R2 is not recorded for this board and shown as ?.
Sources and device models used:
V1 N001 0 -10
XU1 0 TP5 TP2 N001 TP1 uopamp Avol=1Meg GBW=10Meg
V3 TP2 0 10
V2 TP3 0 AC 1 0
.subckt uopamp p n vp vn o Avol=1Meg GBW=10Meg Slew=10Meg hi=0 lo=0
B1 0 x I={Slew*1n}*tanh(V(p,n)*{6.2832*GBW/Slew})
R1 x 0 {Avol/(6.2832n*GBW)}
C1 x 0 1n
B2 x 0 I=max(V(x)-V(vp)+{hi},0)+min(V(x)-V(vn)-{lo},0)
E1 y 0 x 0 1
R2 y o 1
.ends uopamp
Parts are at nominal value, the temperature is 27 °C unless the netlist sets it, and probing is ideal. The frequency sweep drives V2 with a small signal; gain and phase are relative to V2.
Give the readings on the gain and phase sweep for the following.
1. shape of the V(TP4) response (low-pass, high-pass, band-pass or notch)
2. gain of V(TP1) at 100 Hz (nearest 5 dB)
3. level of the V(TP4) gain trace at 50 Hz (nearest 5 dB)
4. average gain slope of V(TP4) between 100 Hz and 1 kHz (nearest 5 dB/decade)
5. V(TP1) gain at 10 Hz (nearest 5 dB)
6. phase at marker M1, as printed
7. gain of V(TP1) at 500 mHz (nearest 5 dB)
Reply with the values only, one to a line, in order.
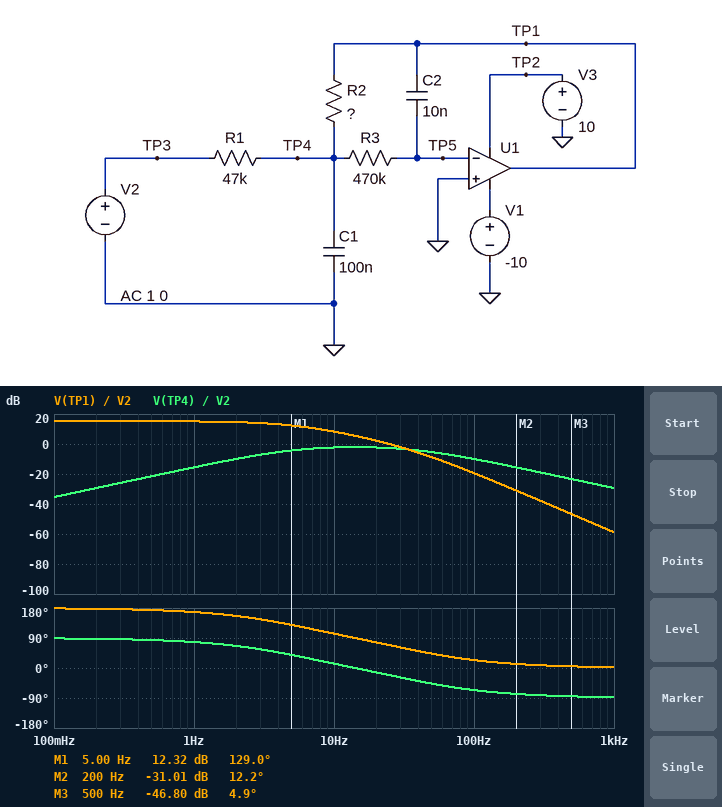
band-pass
-20 dB
-5 dB
-20 dB/decade
10 dB
129.0 deg
15 dB
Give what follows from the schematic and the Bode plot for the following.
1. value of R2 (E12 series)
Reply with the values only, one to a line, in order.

270 kΩ
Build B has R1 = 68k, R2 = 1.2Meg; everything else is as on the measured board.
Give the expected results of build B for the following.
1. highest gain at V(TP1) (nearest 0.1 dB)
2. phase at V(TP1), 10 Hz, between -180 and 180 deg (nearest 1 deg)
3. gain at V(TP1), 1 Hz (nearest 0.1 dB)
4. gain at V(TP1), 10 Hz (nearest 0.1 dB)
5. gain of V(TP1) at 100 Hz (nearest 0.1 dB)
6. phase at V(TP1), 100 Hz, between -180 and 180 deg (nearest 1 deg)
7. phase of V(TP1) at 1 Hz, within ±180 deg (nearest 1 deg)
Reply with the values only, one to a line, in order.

24.9 dB
79 deg
23.6 dB
8.8 dB
-22.3 dB
16 deg
147 deg
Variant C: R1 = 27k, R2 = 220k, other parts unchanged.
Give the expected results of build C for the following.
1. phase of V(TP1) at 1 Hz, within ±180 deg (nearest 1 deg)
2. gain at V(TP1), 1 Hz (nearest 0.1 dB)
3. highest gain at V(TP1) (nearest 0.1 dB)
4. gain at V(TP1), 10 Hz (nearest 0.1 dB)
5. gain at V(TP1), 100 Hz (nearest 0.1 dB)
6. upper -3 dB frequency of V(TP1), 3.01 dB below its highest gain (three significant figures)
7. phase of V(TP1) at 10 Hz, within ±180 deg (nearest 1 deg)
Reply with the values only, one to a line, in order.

164 deg
17.9 dB
18.2 dB
9.0 dB
-15.6 dB
3.71 Hz
102 deg
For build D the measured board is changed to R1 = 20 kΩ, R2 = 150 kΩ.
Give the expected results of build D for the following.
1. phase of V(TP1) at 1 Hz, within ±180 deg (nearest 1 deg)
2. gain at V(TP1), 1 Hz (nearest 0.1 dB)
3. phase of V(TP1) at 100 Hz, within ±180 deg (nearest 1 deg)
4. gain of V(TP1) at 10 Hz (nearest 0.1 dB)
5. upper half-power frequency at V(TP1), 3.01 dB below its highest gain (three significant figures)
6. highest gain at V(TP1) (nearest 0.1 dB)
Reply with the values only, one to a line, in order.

165 deg
17.2 dB
44 deg
8.9 dB
4.00 Hz
17.5 dB
